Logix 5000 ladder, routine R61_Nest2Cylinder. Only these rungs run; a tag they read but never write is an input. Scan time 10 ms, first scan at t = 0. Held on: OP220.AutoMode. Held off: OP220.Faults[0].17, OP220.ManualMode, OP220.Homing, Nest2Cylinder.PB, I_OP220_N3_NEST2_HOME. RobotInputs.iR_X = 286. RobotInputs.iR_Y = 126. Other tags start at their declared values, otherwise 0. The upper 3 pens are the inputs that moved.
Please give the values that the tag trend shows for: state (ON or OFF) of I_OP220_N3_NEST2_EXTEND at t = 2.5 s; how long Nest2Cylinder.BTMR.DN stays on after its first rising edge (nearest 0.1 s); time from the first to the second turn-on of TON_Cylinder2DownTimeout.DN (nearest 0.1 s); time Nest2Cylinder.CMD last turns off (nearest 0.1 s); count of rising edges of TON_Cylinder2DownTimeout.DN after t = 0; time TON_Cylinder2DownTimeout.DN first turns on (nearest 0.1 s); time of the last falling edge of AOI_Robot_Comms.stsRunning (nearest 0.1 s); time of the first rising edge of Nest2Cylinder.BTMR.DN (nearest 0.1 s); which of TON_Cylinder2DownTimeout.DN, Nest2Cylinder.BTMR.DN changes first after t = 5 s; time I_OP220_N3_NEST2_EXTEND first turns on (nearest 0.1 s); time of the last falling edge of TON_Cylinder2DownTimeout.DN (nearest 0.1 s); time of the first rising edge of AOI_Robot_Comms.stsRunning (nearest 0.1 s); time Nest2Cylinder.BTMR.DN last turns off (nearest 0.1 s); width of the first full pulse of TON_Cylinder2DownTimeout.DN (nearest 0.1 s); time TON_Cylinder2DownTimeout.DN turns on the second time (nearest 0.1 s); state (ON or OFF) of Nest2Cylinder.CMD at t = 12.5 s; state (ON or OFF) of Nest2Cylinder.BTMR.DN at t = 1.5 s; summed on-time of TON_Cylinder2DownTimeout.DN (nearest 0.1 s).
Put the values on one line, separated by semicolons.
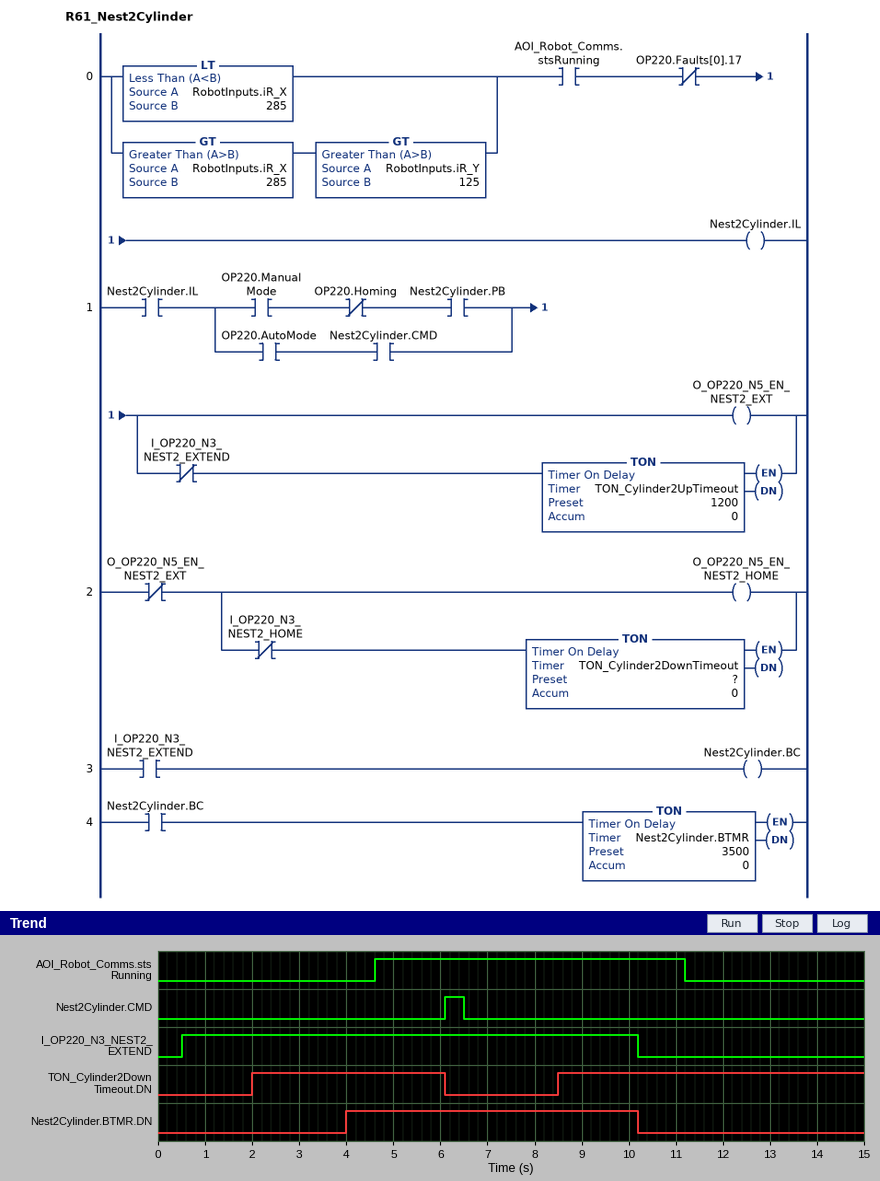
ON; 6.2 s; 6.5 s; 6.5 s; 2; 2.0 s; 11.2 s; 4.0 s; TON_Cylinder2DownTimeout.DN; 0.5 s; 6.1 s; 4.6 s; 10.2 s; 4.1 s; 8.5 s; OFF; OFF; 10.6 s
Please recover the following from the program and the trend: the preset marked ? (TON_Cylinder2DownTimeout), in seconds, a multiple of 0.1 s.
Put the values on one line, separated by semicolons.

2.0 s
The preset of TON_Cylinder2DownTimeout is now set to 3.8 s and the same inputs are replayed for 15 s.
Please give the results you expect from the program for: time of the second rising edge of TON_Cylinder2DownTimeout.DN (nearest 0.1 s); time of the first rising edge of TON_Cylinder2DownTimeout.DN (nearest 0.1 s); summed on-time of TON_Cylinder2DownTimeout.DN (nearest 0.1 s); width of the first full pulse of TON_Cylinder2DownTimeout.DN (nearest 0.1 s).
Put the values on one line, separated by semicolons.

10.3 s; 3.8 s; 7.0 s; 2.3 s
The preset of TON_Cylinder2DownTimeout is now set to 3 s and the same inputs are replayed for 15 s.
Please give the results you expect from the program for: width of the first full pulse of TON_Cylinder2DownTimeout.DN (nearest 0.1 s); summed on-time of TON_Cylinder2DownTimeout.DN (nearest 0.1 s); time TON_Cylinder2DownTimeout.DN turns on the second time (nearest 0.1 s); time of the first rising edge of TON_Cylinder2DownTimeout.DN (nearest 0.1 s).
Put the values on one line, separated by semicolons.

3.1 s; 8.6 s; 9.5 s; 3.0 s
